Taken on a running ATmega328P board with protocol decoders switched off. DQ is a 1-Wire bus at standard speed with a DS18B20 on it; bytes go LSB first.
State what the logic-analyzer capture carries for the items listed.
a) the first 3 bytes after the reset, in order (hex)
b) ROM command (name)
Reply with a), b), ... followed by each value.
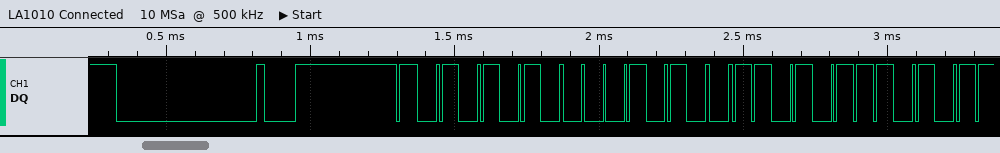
a) 55 28 EB
b) Match ROM
